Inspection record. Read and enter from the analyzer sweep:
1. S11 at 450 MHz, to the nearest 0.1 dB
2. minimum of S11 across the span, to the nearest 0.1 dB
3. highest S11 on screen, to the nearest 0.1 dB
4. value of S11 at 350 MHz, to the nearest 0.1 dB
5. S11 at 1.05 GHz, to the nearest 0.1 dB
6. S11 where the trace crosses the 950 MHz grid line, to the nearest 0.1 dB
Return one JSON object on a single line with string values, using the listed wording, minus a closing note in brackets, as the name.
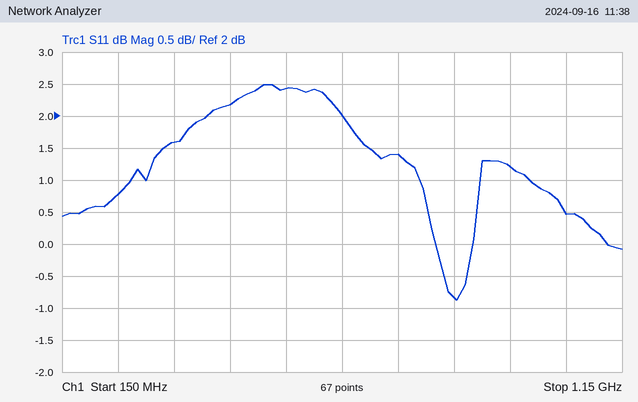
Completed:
{"S11 at 450 MHz, to the nearest 0.1 dB": "2.2 dB", "minimum of S11 across the span, to the nearest 0.1 dB": "-0.9 dB", "highest S11 on screen, to the nearest 0.1 dB": "2.5 dB", "value of S11 at 350 MHz, to the nearest 0.1 dB": "1.6 dB", "S11 at 1.05 GHz, to the nearest 0.1 dB": "0.5 dB", "S11 where the trace crosses the 950 MHz grid line, to the nearest 0.1 dB": "1.2 dB"}
